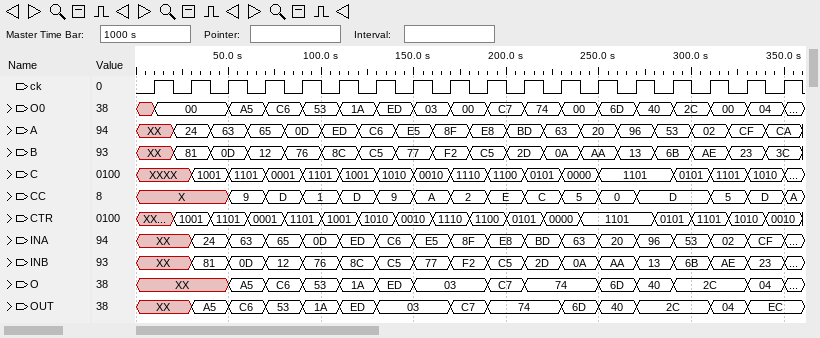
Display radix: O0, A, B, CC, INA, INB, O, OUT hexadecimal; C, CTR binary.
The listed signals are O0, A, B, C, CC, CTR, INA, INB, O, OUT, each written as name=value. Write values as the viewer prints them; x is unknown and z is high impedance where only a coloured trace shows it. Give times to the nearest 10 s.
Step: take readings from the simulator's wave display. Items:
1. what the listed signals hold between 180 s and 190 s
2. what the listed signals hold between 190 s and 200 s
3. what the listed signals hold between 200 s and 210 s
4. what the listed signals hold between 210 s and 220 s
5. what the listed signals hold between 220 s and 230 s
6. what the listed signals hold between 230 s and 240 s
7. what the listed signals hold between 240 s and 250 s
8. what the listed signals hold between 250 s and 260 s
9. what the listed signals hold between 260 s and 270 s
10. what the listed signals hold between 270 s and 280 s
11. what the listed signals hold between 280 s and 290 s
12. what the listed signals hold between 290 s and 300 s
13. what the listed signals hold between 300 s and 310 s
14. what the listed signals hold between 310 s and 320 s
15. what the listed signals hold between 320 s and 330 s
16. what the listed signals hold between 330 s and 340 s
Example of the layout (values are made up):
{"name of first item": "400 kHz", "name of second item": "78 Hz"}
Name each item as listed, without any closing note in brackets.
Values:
{"what the listed signals hold between 180 s and 190 s": "O0=00, A=E8, B=C5, C=1110, CC=2, CTR=1100, INA=8F, INB=F2, O=03, OUT=C7", "what the listed signals hold between 190 s and 200 s": "O0=C7, A=E8, B=C5, C=1100, CC=E, CTR=1100, INA=E8, INB=C5, O=C7, OUT=74", "what the listed signals hold between 200 s and 210 s": "O0=C7, A=BD, B=2D, C=1100, CC=E, CTR=0101, INA=E8, INB=C5, O=C7, OUT=74", "what the listed signals hold between 210 s and 220 s": "O0=74, A=BD, B=2D, C=0101, CC=C, CTR=0101, INA=BD, INB=2D, O=74, OUT=74", "what the listed signals hold between 220 s and 230 s": "O0=74, A=63, B=0A, C=0101, CC=C, CTR=0000, INA=BD, INB=2D, O=74, OUT=74", "what the listed signals hold between 230 s and 240 s": "O0=00, A=63, B=0A, C=0000, CC=5, CTR=0000, INA=63, INB=0A, O=74, OUT=6D", "what the listed signals hold between 240 s and 250 s": "O0=00, A=20, B=AA, C=0000, CC=5, CTR=1101, INA=63, INB=0A, O=74, OUT=6D", "what the listed signals hold between 250 s and 260 s": "O0=6D, A=20, B=AA, C=1101, CC=0, CTR=1101, INA=20, INB=AA, O=6D, OUT=40", "what the listed signals hold between 260 s and 270 s": "O0=6D, A=96, B=13, C=1101, CC=0, CTR=1101, INA=20, INB=AA, O=6D, OUT=40", "what the listed signals hold between 270 s and 280 s": "O0=40, A=96, B=13, C=1101, CC=D, CTR=1101, INA=96, INB=13, O=40, OUT=2C", "what the listed signals hold between 280 s and 290 s": "O0=40, A=53, B=6B, C=1101, CC=D, CTR=0101, INA=96, INB=13, O=40, OUT=2C", "what the listed signals hold between 290 s and 300 s": "O0=2C, A=53, B=6B, C=0101, CC=D, CTR=0101, INA=53, INB=6B, O=2C, OUT=2C", "what the listed signals hold between 300 s and 310 s": "O0=2C, A=02, B=AE, C=0101, CC=D, CTR=1101, INA=53, INB=6B, O=2C, OUT=2C", "what the listed signals hold between 310 s and 320 s": "O0=00, A=02, B=AE, C=1101, CC=5, CTR=1101, INA=02, INB=AE, O=2C, OUT=04", "what the listed signals hold between 320 s and 330 s": "O0=00, A=CF, B=23, C=1101, CC=5, CTR=1010, INA=02, INB=AE, O=2C, OUT=04", "what the listed signals hold between 330 s and 340 s": "O0=04, A=CF, B=23, C=1010, CC=D, CTR=1010, INA=CF, INB=23, O=04, OUT=EC"}
